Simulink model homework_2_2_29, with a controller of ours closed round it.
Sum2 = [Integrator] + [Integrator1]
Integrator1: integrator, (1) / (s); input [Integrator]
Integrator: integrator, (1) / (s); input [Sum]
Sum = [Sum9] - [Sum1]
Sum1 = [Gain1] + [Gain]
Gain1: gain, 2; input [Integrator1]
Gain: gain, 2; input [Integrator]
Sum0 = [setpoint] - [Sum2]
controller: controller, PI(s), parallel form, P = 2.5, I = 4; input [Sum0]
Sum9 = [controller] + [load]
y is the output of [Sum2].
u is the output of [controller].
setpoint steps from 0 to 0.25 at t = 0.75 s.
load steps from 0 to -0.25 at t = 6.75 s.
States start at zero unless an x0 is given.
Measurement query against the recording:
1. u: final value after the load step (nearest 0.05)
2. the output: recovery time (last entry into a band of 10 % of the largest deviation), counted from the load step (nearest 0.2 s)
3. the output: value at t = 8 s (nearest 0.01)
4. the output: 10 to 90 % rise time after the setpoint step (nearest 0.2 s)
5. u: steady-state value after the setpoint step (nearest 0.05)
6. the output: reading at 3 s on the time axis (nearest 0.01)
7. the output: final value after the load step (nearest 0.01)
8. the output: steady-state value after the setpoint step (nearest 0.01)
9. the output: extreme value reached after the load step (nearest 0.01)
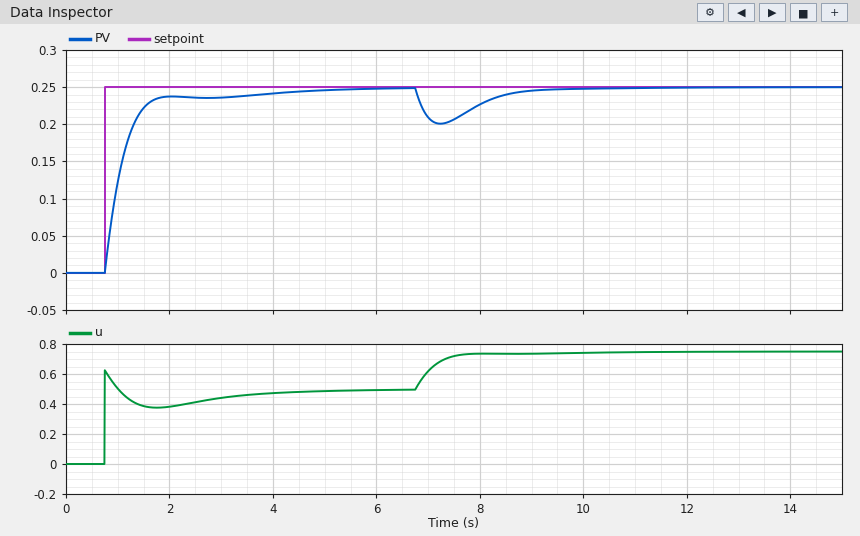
0.75
2.2 s
0.23
0.8 s
0.50
0.24
0.25
0.25
0.20
